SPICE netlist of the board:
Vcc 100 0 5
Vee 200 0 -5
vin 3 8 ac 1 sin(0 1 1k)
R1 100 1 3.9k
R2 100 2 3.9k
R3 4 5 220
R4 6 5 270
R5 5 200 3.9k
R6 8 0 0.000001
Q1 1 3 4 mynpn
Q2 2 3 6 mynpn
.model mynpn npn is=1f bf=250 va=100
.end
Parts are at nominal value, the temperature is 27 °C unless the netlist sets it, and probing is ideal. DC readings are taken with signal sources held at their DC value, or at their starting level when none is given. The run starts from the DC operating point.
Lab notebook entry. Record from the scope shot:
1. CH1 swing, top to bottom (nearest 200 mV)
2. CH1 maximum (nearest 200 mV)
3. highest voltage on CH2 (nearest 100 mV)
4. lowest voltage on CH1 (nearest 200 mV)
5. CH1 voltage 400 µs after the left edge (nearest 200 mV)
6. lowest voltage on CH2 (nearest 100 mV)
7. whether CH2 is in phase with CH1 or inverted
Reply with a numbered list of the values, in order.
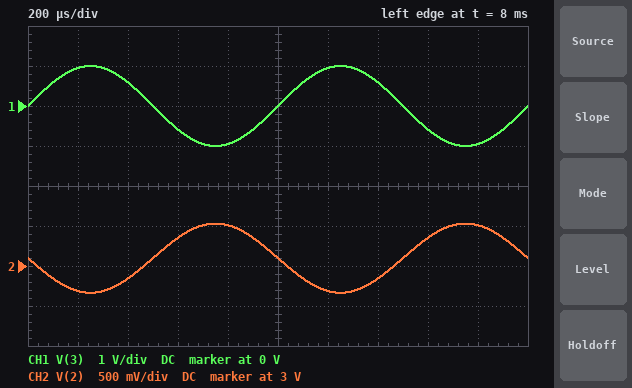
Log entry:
1. 2.0 V
2. 1.0 V
3. 3.5 V
4. -1.0 V
5. 600 mV
6. 2.7 V
7. inverted
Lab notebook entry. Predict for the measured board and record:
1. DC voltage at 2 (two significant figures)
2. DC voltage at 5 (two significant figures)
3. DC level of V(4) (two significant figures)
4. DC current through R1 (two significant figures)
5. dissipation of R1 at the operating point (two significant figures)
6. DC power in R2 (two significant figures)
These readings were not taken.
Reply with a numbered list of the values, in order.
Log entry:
1. 3.1 V
2. -830 mV
3. -700 mV
4. 580 µA
5. 1.3 mW
6. 930 µW
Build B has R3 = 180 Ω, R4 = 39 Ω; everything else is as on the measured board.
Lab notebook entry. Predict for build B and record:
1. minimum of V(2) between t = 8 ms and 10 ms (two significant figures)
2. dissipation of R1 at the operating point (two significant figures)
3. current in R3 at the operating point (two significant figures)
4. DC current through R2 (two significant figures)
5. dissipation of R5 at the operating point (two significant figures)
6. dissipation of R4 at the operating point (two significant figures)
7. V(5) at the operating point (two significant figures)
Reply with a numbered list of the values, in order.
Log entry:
1. 1.2 V
2. 370 µW
3. 310 µA
4. 780 µA
5. 4.7 mW
6. 24 µW
7. -740 mV
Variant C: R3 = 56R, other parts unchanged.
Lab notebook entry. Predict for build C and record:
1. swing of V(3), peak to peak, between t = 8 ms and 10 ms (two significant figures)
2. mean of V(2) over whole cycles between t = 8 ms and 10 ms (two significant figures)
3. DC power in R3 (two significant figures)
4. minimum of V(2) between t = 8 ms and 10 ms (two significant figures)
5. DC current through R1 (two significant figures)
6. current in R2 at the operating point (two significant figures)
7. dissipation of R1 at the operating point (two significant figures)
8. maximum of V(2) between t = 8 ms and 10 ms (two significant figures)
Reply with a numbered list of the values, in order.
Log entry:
1. 2.0 V
2. 3.9 V
3. 37 µW
4. 3.7 V
5. 810 µA
6. 270 µA
7. 2.6 mW
8. 4.1 V
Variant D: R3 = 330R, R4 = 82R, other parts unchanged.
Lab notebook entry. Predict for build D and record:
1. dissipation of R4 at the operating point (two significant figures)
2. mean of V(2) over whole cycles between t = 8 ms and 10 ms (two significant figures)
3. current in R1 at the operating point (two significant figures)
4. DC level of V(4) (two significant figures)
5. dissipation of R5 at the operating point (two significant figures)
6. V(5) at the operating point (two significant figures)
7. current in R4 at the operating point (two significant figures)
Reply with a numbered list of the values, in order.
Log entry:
1. 53 µW
2. 1.9 V
3. 280 µA
4. -680 mV
5. 4.6 mW
6. -770 mV
7. 800 µA
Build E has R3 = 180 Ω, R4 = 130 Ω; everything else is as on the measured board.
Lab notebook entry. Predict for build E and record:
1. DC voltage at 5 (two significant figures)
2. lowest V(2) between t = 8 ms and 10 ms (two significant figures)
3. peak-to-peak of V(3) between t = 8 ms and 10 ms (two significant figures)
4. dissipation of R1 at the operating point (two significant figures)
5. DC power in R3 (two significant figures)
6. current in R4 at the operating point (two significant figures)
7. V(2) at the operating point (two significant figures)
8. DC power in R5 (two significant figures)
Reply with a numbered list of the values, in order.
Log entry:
1. -780 mV
2. 2.1 V
3. 2.0 V
4. 870 µW
5. 41 µW
6. 610 µA
7. 2.6 V
8. 4.6 mW
